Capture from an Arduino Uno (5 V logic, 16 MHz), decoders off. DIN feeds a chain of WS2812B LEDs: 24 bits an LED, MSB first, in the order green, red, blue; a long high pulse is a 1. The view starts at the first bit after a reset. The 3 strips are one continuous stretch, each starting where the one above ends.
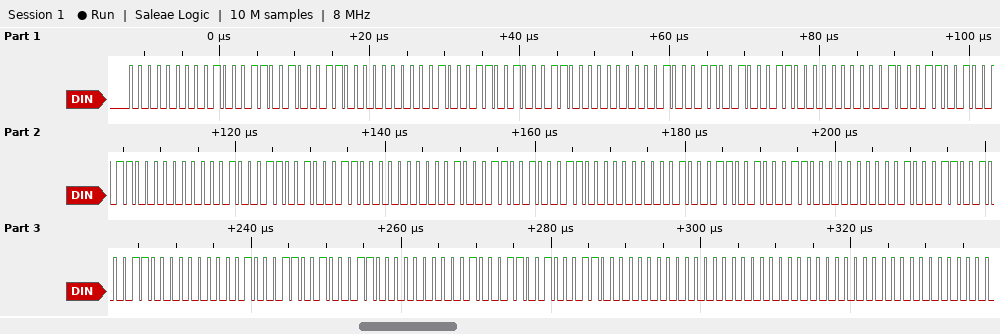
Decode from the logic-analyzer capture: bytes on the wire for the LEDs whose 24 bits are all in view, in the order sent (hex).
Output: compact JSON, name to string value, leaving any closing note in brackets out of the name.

{"bytes on the wire for the LEDs whose 24 bits are all in view, in the order sent": "00 46 46 00 46 46 00 46 46 00 46 46 00 46 46 00 46 46 00 46 46 00 46 46 00 46 46 00 46 46 00 00 00"}
